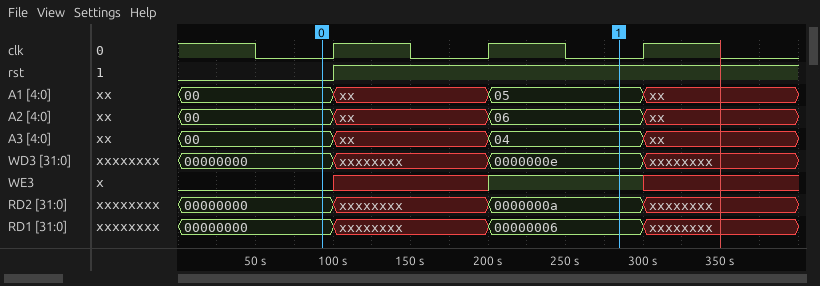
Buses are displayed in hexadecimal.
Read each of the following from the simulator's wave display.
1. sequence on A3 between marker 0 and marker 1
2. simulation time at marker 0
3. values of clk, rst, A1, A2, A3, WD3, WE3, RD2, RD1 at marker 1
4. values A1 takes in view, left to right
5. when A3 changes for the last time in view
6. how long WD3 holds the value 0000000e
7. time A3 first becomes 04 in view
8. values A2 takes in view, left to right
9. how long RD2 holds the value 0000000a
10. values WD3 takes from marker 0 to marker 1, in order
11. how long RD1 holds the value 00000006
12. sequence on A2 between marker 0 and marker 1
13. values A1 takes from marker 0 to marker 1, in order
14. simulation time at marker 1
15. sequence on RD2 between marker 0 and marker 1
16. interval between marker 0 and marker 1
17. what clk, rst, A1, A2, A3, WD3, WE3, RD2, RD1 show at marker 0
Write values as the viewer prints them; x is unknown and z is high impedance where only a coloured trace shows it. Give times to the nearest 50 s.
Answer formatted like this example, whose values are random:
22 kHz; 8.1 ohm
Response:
00, xx, 04; 100 s; clk=0, rst=1, A1=05, A2=06, A3=04, WD3=0000000e, WE3=1, RD2=0000000a, RD1=00000006; 00, xx, 05, xx; 300 s; 100 s; 200 s; 00, xx, 06, xx; 100 s; 00000000, xxxxxxxx, 0000000e; 100 s; 00, xx, 06; 00, xx, 05; 300 s; 00000000, xxxxxxxx, 0000000a; 200 s; clk=0, rst=0, A1=00, A2=00, A3=00, WD3=00000000, WE3=0, RD2=00000000, RD1=00000000
